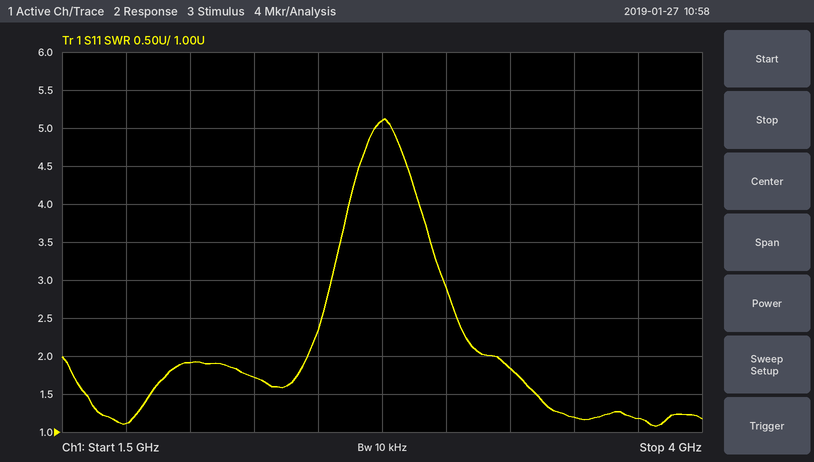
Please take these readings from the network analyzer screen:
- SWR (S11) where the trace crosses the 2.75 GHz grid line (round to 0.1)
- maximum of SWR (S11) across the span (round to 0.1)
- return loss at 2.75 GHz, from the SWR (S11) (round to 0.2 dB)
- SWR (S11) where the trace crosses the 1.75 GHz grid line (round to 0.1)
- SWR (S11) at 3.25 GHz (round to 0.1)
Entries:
5.1
5.1
3.4 dB
1.1
1.8
